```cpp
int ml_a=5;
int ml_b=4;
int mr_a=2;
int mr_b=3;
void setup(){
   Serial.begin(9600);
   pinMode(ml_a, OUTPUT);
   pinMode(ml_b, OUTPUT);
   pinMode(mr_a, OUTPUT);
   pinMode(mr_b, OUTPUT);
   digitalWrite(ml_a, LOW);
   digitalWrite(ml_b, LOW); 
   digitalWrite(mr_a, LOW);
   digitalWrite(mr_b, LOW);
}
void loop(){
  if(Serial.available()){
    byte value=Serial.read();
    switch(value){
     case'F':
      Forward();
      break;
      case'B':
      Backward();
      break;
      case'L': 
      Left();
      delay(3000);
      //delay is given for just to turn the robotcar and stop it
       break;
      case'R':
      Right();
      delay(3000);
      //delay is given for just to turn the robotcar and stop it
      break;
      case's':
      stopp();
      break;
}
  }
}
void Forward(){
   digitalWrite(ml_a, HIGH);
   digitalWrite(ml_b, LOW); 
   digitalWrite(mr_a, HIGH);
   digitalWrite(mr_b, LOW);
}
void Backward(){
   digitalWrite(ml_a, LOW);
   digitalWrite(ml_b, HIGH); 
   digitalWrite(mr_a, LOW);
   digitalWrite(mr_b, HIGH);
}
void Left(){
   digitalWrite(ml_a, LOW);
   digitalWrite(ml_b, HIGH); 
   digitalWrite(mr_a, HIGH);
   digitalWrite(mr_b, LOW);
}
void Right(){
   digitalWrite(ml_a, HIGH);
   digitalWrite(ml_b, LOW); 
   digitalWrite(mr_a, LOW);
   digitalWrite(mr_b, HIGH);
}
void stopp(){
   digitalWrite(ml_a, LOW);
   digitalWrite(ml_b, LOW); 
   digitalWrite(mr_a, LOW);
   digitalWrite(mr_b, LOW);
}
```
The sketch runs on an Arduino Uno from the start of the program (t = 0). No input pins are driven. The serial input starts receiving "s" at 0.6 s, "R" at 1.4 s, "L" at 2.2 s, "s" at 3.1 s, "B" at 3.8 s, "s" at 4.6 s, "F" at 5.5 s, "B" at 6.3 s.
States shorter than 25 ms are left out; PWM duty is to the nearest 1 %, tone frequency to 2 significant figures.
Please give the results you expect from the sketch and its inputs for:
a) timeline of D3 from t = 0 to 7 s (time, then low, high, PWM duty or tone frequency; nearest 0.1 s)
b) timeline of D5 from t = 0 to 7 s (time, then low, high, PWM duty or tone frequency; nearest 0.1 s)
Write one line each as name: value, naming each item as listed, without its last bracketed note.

timeline of D3 from t = 0 to 7 s: 0 s low; 1.4 s high; 4.4 s low
timeline of D5 from t = 0 to 7 s: 0 s low; 1.4 s high; 4.4 s low
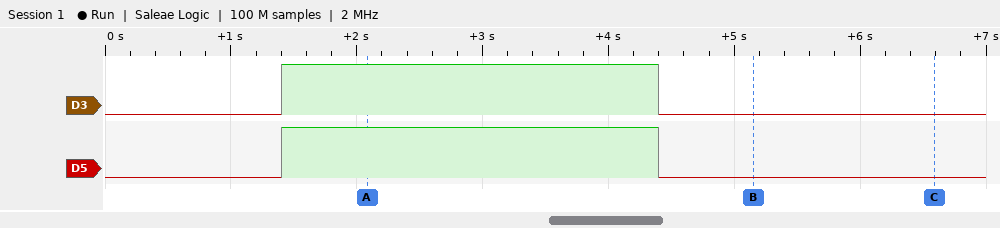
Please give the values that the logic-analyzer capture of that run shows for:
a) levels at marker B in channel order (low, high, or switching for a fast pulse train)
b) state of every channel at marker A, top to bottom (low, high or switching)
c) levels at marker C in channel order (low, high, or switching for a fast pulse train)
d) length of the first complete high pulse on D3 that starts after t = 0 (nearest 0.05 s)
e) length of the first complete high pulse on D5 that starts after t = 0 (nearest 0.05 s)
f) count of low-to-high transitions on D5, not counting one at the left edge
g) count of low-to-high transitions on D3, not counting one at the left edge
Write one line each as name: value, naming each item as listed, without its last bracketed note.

levels at marker B in channel order: D3 low, D5 low
state of every channel at marker A, top to bottom: D3 high, D5 high
levels at marker C in channel order: D3 low, D5 low
length of the first complete high pulse on D3 that starts after t = 0: 3.00 s
length of the first complete high pulse on D5 that starts after t = 0: 3.00 s
count of low-to-high transitions on D5, not counting one at the left edge: 1
count of low-to-high transitions on D3, not counting one at the left edge: 1
